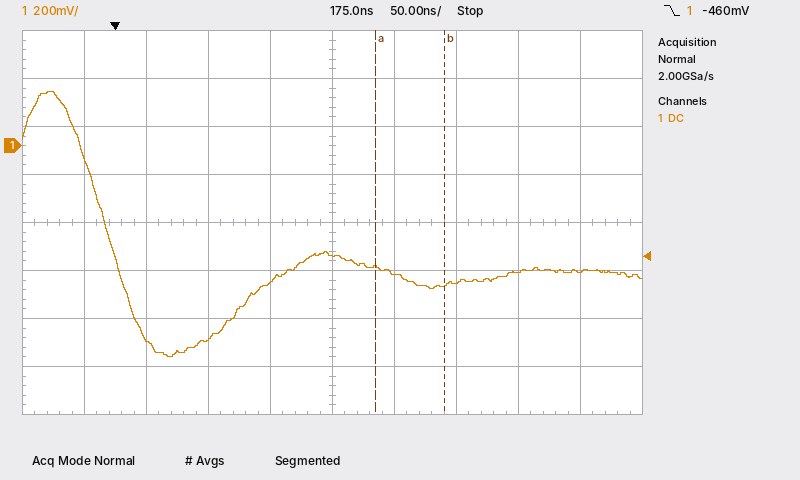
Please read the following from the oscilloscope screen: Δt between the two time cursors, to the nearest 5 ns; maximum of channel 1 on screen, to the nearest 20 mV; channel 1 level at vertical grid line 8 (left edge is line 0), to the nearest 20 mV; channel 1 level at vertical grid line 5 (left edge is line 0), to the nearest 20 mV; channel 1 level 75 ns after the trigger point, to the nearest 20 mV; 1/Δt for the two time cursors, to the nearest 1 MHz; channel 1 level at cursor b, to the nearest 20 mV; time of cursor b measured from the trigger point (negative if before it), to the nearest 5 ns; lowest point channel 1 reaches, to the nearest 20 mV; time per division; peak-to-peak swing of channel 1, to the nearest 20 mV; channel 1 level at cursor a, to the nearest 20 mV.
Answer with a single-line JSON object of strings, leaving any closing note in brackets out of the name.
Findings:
{"Δt between the two time cursors, to the nearest 5 ns": "55 ns", "maximum of channel 1 on screen, to the nearest 20 mV": "220 mV", "channel 1 level at vertical grid line 8 (left edge is line 0), to the nearest 20 mV": "-520 mV", "channel 1 level at vertical grid line 5 (left edge is line 0), to the nearest 20 mV": "-460 mV", "channel 1 level 75 ns after the trigger point, to the nearest 20 mV": "-800 mV", "1/Δt for the two time cursors, to the nearest 1 MHz": "18 MHz", "channel 1 level at cursor b, to the nearest 20 mV": "-580 mV", "time of cursor b measured from the trigger point (negative if before it), to the nearest 5 ns": "+265 ns", "lowest point channel 1 reaches, to the nearest 20 mV": "-880 mV", "time per division": "50 ns", "peak-to-peak swing of channel 1, to the nearest 20 mV": "1.10 V", "channel 1 level at cursor a, to the nearest 20 mV": "-500 mV"}
